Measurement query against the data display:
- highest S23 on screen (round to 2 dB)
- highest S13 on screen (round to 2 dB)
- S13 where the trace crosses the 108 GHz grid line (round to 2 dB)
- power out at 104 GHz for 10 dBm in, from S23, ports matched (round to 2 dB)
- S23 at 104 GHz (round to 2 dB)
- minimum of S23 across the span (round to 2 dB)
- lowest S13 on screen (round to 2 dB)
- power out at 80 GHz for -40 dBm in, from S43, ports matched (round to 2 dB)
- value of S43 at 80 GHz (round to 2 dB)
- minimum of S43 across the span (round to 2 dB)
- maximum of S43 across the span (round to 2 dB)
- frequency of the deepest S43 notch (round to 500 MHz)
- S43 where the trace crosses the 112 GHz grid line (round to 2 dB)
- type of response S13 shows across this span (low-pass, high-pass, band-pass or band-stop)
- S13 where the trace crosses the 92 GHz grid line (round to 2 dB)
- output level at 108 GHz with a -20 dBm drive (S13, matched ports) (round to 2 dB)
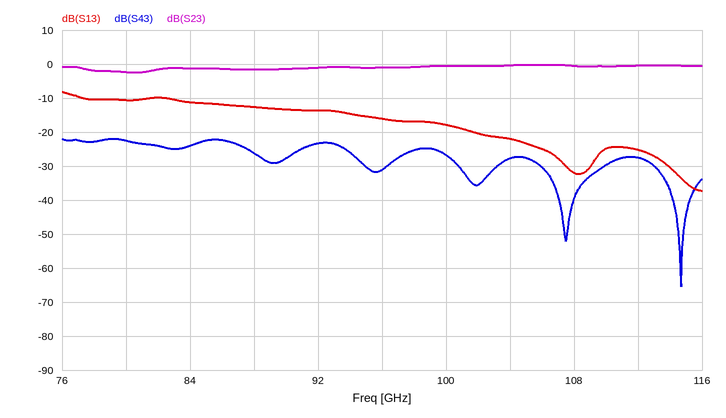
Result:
0 dB
-8 dB
-32 dB
10 dBm
0 dB
-2 dB
-38 dB
-62 dBm
-22 dB
-66 dB
-22 dB
114.5 GHz
-28 dB
low-pass
-14 dB
-52 dBm
